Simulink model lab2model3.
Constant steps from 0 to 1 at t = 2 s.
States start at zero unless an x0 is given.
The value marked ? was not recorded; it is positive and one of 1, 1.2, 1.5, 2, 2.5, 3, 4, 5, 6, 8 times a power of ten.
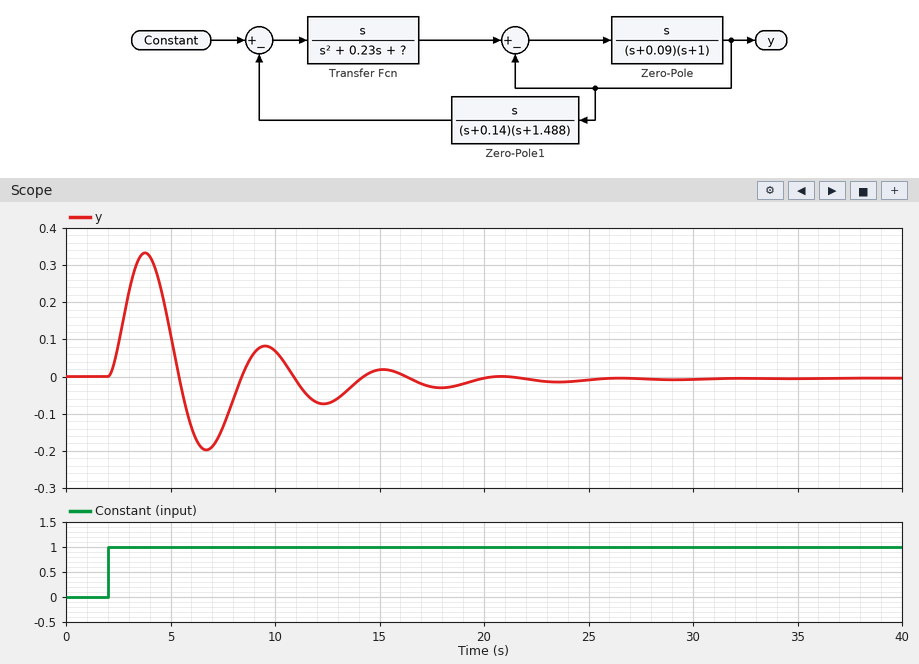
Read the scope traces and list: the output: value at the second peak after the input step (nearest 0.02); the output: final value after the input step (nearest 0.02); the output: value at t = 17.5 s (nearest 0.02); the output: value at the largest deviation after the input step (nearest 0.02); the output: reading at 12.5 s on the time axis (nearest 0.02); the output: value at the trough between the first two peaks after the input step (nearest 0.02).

0.08
0.00
-0.02
0.34
-0.08
-0.20
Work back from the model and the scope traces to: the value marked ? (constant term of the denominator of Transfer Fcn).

1
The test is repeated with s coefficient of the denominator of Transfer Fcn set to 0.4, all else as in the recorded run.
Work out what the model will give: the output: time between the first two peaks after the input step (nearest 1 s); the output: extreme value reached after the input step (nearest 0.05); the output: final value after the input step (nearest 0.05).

6 s
0.30
0.00
